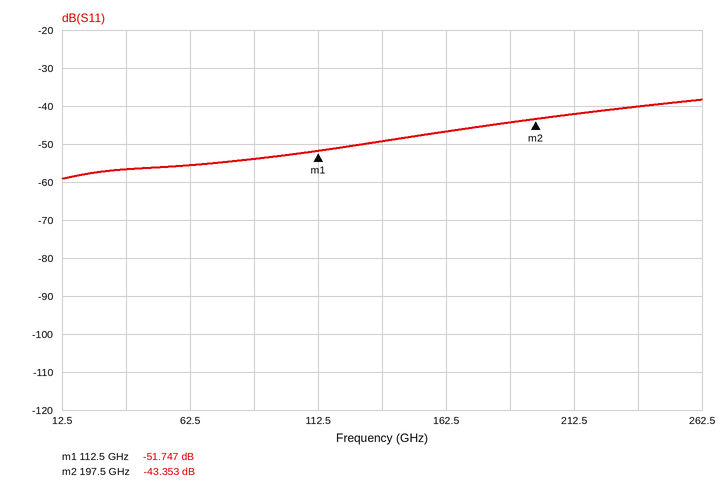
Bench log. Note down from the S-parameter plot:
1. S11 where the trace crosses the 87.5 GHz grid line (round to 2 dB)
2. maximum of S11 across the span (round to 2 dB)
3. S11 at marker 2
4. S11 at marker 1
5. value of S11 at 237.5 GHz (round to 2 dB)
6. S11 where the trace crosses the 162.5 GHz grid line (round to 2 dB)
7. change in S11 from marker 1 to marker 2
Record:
-54 dB
-38 dB
-43.353 dB
-51.747 dB
-40 dB
-46 dB
8.394 dB
